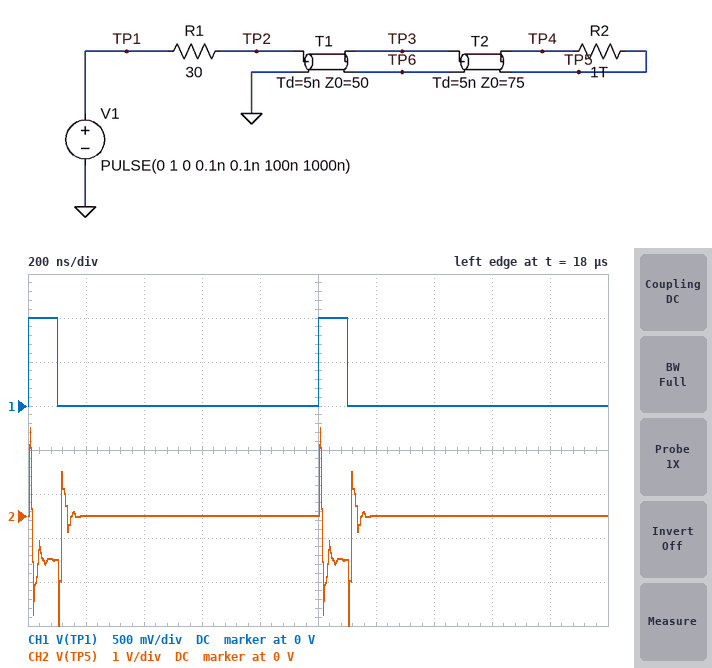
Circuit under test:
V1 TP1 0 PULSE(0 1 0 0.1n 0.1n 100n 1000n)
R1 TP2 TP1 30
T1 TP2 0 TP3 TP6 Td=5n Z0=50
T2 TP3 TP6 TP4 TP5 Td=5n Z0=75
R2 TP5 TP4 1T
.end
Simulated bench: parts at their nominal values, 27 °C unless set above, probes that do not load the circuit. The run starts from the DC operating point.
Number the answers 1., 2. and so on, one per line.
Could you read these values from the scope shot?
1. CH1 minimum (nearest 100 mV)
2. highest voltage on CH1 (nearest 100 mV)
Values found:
1. 0 V
2. 1.0 V
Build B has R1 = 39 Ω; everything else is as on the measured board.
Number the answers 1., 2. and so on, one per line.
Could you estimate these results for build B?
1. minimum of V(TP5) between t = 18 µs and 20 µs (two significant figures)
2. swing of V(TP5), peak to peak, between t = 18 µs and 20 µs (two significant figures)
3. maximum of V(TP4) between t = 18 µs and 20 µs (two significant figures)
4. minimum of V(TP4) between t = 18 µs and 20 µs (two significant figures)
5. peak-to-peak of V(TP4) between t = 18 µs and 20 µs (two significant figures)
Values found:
1. -2.8 V
2. 4.6 V
3. 1.8 V
4. -1.8 V
5. 3.6 V
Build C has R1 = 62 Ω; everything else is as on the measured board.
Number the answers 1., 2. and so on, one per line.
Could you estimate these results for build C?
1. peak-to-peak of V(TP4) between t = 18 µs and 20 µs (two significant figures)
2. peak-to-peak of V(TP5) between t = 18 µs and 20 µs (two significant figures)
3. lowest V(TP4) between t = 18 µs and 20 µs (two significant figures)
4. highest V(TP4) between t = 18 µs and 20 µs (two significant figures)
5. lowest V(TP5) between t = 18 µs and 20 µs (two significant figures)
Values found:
1. 2.8 V
2. 3.8 V
3. -1.4 V
4. 1.4 V
5. -2.4 V
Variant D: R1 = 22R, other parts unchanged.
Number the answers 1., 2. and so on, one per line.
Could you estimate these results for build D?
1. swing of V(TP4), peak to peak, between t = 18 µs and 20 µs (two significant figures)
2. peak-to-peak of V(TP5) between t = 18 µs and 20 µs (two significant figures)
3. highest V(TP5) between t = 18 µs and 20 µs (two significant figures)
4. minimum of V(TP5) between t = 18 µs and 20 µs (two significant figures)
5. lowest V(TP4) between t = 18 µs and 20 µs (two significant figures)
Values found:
1. 4.4 V
2. 5.4 V
3. 2.2 V
4. -3.2 V
5. -2.2 V
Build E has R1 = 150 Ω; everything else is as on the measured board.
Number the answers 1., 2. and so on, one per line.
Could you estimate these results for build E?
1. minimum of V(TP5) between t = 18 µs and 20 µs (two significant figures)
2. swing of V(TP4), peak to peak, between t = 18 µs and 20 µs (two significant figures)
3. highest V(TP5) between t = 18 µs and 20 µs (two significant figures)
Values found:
1. -1.8 V
2. 1.6 V
3. 800 mV
